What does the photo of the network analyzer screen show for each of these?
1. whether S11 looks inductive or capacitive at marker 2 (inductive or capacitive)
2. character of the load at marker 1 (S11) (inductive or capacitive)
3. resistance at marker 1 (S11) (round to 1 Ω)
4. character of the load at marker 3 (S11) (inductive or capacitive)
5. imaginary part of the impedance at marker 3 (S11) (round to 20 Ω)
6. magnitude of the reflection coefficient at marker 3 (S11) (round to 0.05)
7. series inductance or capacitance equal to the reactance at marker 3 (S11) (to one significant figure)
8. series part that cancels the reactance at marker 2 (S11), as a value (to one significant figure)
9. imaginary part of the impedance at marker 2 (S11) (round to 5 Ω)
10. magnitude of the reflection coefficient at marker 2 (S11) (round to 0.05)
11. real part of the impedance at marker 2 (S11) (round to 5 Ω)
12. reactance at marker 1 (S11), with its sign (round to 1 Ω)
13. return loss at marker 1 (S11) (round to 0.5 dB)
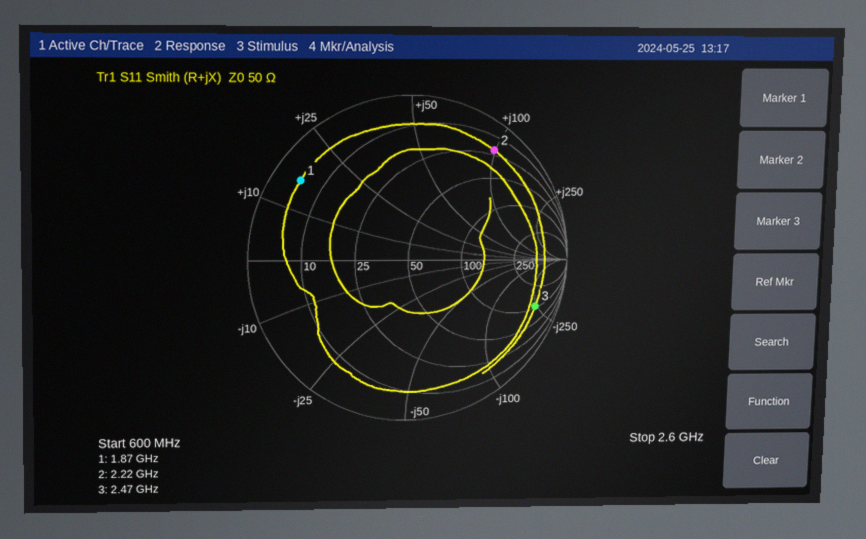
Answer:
inductive
inductive
5 Ω
capacitive
-240 Ω
0.85
300 fF
700 fF
+100 Ω
0.85
20 Ω
+16 Ω
1.5 dB
